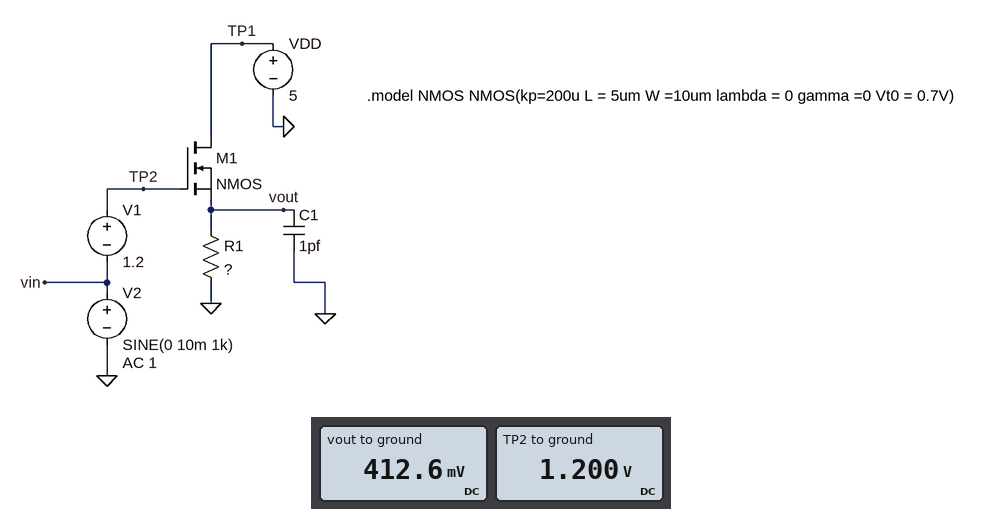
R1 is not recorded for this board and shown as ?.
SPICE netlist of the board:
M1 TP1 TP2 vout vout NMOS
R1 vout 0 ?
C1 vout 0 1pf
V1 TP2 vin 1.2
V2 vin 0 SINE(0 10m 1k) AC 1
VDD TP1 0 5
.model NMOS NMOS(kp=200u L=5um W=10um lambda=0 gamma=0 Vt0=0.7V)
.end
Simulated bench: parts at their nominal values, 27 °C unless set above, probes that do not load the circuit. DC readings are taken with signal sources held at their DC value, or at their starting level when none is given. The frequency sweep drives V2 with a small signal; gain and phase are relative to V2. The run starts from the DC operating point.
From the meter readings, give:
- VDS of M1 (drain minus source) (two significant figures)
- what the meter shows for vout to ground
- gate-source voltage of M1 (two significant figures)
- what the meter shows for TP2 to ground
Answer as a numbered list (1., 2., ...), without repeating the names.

1. 4.6 V
2. 412.6 mV
3. 790 mV
4. 1.200 V
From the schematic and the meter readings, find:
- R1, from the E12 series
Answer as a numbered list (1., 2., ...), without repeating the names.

1. 270 kΩ
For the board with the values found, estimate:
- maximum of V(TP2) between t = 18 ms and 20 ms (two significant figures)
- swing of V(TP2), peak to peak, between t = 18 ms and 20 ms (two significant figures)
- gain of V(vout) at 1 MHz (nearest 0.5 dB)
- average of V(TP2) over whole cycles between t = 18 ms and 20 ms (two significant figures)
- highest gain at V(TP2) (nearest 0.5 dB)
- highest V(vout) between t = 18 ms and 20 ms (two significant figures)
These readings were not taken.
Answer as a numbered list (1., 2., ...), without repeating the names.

1. 1.2 V
2. 20 mV
3. -1.0 dB
4. 1.2 V
5. 0 dB
6. 420 mV
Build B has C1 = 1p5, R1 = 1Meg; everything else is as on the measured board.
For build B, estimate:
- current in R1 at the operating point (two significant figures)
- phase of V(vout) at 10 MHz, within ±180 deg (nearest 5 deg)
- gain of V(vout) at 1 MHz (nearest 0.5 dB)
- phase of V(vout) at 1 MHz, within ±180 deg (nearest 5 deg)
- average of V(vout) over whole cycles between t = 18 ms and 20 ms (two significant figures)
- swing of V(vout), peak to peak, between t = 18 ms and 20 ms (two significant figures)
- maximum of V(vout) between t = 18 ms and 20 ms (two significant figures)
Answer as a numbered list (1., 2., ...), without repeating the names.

1. 450 nA
2. -80 deg
3. -1.5 dB
4. -25 deg
5. 450 mV
6. 19 mV
7. 460 mV
